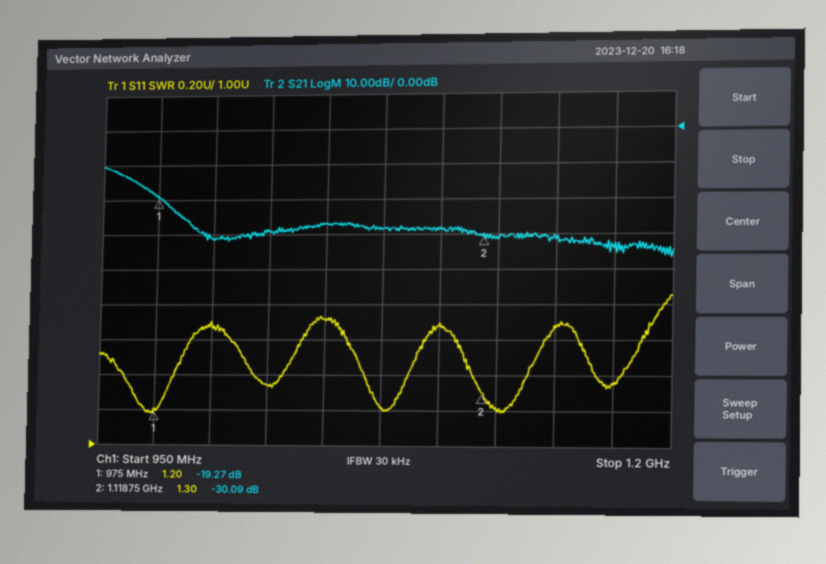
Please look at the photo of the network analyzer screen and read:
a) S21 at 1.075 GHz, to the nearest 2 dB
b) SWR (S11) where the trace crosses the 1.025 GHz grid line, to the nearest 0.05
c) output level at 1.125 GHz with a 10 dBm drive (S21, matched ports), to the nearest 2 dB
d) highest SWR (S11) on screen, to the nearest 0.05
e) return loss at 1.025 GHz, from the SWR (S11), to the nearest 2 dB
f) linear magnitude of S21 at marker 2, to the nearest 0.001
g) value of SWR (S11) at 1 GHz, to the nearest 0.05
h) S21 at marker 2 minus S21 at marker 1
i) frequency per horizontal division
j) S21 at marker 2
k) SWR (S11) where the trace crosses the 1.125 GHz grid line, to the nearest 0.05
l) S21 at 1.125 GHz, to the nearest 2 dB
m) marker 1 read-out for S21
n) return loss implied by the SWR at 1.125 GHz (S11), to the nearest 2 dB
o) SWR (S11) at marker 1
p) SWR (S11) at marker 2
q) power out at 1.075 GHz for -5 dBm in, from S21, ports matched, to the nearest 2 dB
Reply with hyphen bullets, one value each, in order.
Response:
- -28 dB
- 1.35
- -22 dBm
- 1.85
- 16 dB
- 0.031
- 1.70
- -10.82 dB
- 25 MHz
- -30.09 dB
- 1.20
- -32 dB
- -19.27 dB
- 20 dB
- 1.20
- 1.30
- -34 dBm
